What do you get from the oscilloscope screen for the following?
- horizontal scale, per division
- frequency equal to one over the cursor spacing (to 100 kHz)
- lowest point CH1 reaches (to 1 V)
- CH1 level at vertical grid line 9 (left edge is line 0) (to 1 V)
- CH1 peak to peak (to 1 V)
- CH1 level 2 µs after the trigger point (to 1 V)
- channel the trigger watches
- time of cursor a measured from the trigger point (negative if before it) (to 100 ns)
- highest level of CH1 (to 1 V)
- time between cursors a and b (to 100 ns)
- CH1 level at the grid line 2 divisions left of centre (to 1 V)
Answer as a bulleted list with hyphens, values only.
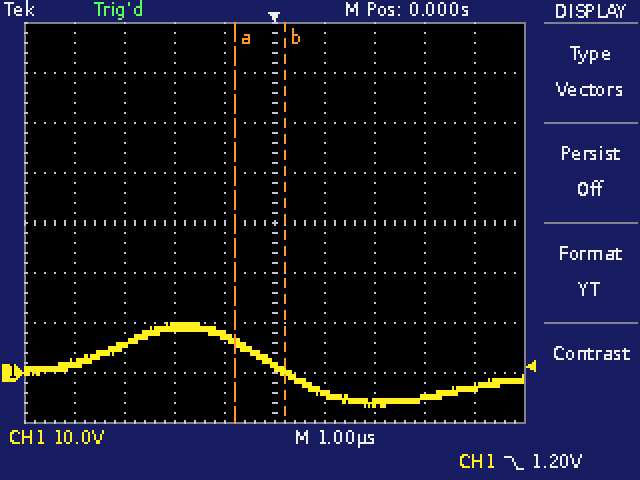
- 1 µs
- 1.0 MHz
- -7 V
- -3 V
- 17 V
- -6 V
- CH1
- -800 ns
- 10 V
- 1.0 µs
- 9 V
